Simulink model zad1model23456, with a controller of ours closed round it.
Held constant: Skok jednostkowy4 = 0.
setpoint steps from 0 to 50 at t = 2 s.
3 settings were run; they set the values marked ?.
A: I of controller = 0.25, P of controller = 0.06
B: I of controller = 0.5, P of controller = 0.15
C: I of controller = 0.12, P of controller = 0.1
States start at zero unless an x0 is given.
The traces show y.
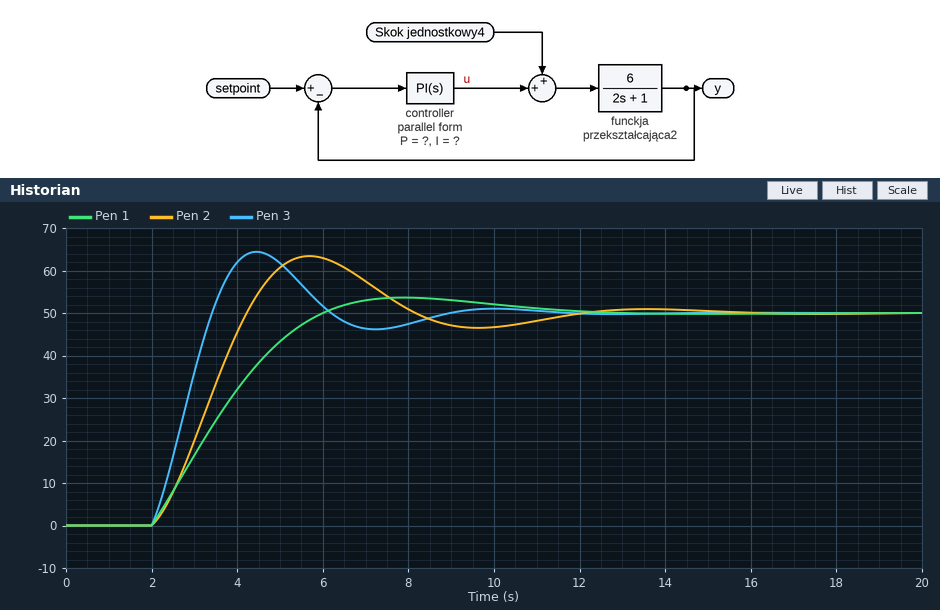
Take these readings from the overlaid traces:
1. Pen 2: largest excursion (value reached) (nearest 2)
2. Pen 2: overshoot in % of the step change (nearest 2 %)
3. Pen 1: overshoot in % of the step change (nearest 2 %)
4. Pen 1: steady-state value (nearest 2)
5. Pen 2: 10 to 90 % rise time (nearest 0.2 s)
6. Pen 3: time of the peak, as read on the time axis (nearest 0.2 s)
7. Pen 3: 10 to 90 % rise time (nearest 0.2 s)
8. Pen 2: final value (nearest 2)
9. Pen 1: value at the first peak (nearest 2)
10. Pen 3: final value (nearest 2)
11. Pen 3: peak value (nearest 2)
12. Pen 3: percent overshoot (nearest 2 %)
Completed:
64
26 %
8 %
50
1.6 s
4.4 s
1.0 s
50
54
50
64
28 %
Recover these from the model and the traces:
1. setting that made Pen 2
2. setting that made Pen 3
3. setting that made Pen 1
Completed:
A
B
C
